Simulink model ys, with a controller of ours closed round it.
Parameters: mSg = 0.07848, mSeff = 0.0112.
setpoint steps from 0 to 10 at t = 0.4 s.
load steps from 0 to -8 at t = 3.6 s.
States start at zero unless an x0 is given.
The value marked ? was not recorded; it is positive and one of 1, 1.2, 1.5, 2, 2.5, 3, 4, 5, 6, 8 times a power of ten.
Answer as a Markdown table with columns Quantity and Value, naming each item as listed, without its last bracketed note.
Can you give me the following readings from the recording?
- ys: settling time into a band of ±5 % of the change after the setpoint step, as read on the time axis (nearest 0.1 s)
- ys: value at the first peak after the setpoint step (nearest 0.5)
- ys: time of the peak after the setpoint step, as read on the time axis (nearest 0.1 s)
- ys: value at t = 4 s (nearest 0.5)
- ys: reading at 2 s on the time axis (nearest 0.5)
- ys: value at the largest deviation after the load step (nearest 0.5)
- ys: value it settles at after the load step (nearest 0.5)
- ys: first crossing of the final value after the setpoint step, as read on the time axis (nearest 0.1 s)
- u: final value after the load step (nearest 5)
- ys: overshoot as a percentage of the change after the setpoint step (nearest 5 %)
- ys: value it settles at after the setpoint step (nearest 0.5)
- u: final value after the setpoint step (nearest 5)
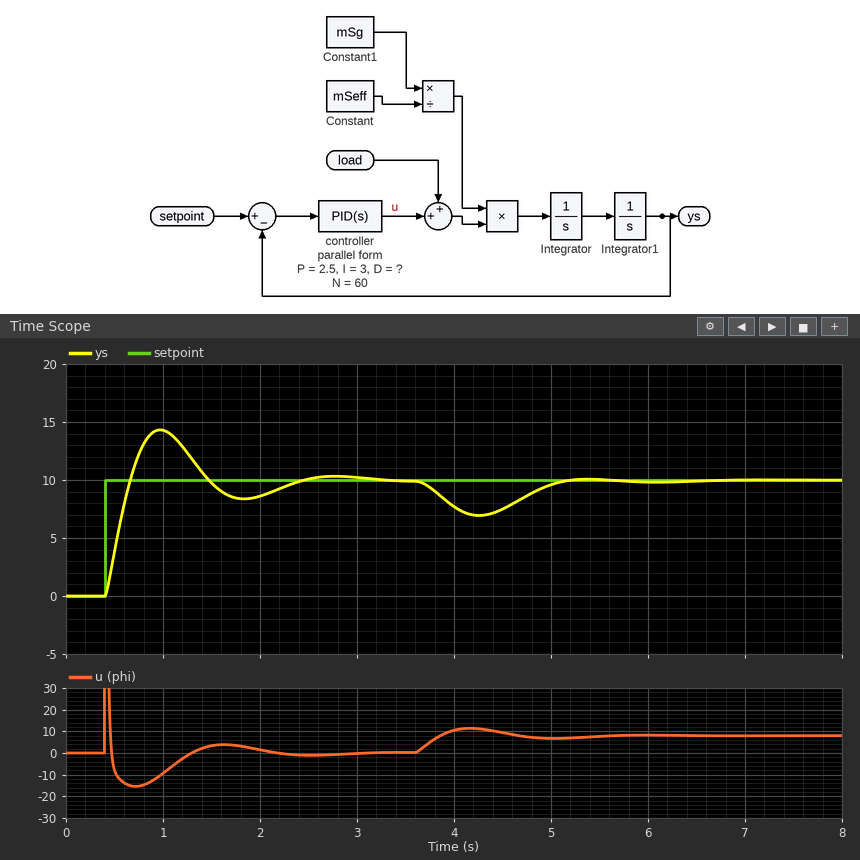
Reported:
| Quantity | Value |
|---|---|
| ys: settling time into a band of ±5 % of the change after the setpoint step, as read on the time axis | 2.3 s |
| ys: value at the first peak after the setpoint step | 14.5 |
| ys: time of the peak after the setpoint step, as read on the time axis | 1.0 s |
| ys: value at t = 4 s | 7.5 |
| ys: reading at 2 s on the time axis | 8.5 |
| ys: value at the largest deviation after the load step | 7.0 |
| ys: value it settles at after the load step | 10.0 |
| ys: first crossing of the final value after the setpoint step, as read on the time axis | 0.7 s |
| u: final value after the load step | 10 |
| ys: overshoot as a percentage of the change after the setpoint step | 45 % |
| ys: value it settles at after the setpoint step | 10.0 |
| u: final value after the setpoint step | 0 |
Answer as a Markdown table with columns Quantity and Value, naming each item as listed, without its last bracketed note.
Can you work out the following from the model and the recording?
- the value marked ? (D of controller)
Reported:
| Quantity | Value |
|---|---|
| the value marked ? | 0.6 |
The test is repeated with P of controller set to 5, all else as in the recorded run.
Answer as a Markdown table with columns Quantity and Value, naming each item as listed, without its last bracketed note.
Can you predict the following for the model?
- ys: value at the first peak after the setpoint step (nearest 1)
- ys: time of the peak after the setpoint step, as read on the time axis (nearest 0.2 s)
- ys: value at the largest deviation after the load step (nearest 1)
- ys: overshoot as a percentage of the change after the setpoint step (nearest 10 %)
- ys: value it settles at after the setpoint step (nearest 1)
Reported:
| Quantity | Value |
|---|---|
| ys: value at the first peak after the setpoint step | 15 |
| ys: time of the peak after the setpoint step, as read on the time axis | 0.8 s |
| ys: value at the largest deviation after the load step | 8 |
| ys: overshoot as a percentage of the change after the setpoint step | 50 % |
| ys: value it settles at after the setpoint step | 10 |
